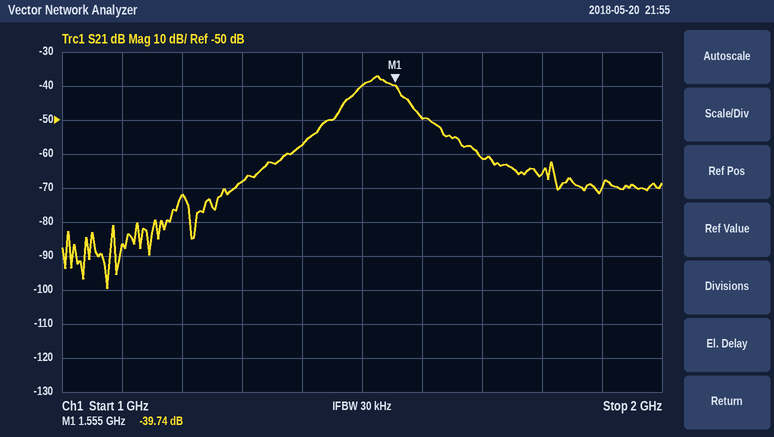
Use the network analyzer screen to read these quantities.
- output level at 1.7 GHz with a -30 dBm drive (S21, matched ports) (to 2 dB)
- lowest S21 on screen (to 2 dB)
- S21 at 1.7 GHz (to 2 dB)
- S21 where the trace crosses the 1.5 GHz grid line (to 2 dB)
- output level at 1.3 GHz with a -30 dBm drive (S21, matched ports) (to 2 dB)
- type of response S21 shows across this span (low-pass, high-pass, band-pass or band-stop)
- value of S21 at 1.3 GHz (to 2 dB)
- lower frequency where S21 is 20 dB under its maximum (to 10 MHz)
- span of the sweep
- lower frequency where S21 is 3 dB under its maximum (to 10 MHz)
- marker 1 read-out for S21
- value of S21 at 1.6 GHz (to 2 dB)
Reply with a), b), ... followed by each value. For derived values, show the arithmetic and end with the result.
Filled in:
a) -30 dBm + (-62 dB) = -92 dBm
b) -100 dB
c) -62 dB
d) -40 dB
e) -30 dBm + (-68 dB) = -98 dBm
f) band-pass
g) -68 dB
h) 1.40 GHz
i) 1 GHz
j) 1.50 GHz
k) -39.74 dB
l) -50 dB
